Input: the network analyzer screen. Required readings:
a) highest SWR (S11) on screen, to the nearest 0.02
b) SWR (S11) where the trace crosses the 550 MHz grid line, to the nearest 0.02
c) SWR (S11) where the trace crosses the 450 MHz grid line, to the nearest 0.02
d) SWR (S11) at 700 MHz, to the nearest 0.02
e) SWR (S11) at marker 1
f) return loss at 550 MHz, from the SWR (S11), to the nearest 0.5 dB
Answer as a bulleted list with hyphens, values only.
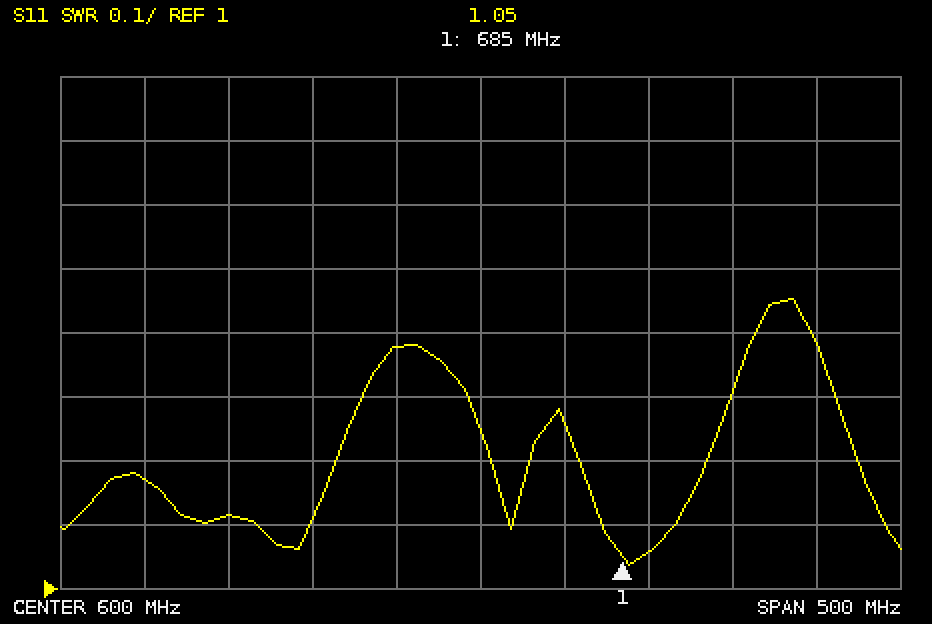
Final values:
- 1.46
- 1.38
- 1.12
- 1.06
- 1.05
- 16.0 dB
